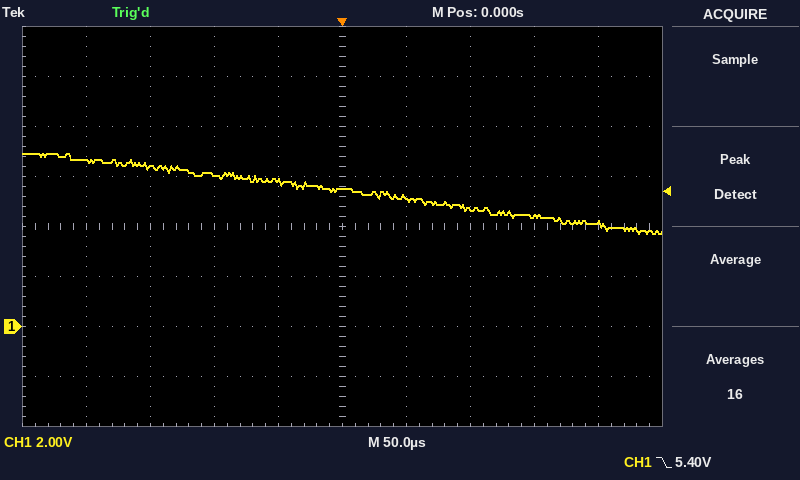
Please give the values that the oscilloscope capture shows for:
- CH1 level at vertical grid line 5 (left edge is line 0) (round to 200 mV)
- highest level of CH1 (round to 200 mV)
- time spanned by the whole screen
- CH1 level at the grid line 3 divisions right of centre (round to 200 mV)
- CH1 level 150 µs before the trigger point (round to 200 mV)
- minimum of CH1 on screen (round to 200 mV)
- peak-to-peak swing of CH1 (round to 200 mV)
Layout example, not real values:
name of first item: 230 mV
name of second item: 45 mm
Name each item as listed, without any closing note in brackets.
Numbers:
CH1 level at vertical grid line 5 (left edge is line 0): 5.6 V
highest level of CH1: 7.0 V
time spanned by the whole screen: 500 µs
CH1 level at the grid line 3 divisions right of centre: 4.4 V
CH1 level 150 µs before the trigger point: 6.4 V
minimum of CH1 on screen: 3.8 V
peak-to-peak swing of CH1: 3.2 V
